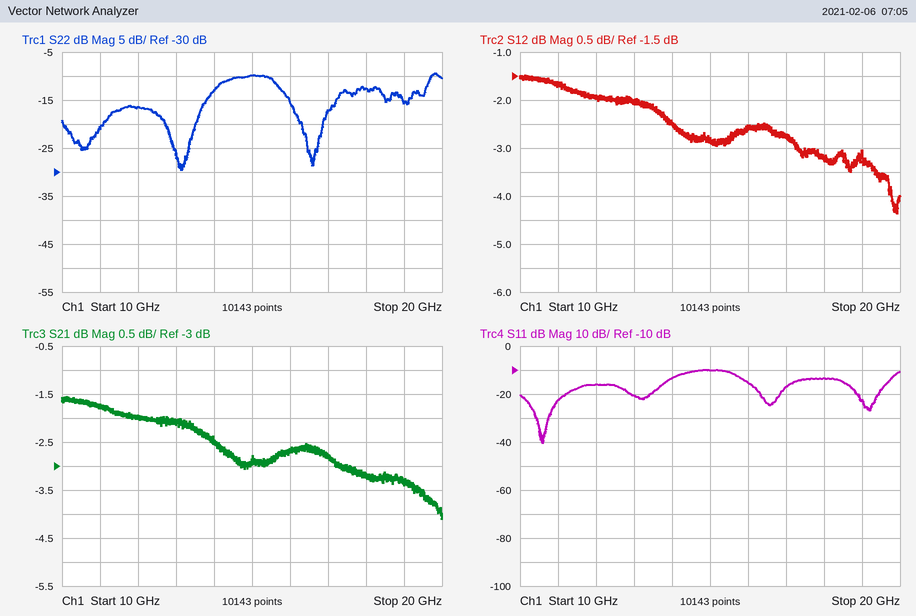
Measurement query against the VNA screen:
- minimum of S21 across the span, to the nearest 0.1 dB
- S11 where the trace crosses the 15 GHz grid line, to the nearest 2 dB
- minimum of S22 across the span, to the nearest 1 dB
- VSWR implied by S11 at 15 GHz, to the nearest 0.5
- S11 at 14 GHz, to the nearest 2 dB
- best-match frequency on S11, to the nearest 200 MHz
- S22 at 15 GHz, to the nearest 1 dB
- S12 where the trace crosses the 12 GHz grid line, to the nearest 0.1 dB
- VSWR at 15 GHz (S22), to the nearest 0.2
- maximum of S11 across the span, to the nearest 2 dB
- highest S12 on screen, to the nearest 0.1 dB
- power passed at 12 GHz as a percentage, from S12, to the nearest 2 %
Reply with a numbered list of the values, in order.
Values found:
1. -4.1 dB
2. -10 dB
3. -30 dB
4. 2.0
5. -14 dB
6. 10.6 GHz
7. -10 dB
8. -1.9 dB
9. 2.0
10. -10 dB
11. -1.5 dB
12. 64 %
